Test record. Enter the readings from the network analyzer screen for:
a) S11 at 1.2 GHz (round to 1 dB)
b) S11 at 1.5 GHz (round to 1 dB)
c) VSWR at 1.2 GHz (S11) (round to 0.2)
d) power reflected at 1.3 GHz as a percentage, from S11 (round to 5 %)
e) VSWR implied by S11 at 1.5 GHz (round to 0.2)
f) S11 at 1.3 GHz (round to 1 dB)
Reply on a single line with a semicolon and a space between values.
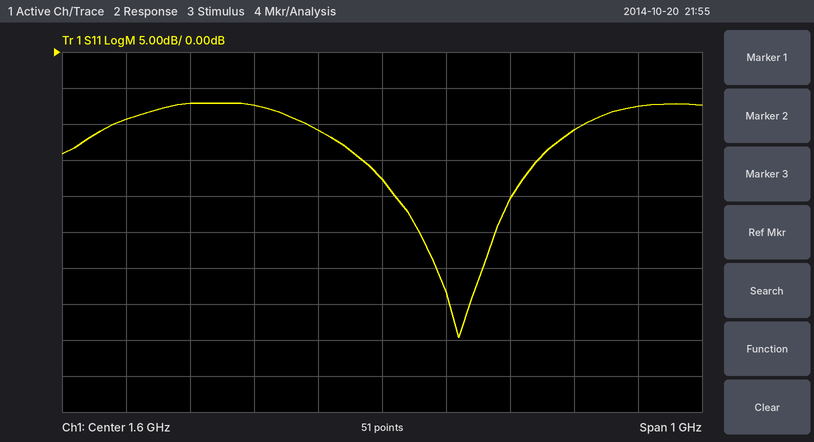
-9 dB; -11 dB; 2.0; 20 %; 1.8; -7 dB
